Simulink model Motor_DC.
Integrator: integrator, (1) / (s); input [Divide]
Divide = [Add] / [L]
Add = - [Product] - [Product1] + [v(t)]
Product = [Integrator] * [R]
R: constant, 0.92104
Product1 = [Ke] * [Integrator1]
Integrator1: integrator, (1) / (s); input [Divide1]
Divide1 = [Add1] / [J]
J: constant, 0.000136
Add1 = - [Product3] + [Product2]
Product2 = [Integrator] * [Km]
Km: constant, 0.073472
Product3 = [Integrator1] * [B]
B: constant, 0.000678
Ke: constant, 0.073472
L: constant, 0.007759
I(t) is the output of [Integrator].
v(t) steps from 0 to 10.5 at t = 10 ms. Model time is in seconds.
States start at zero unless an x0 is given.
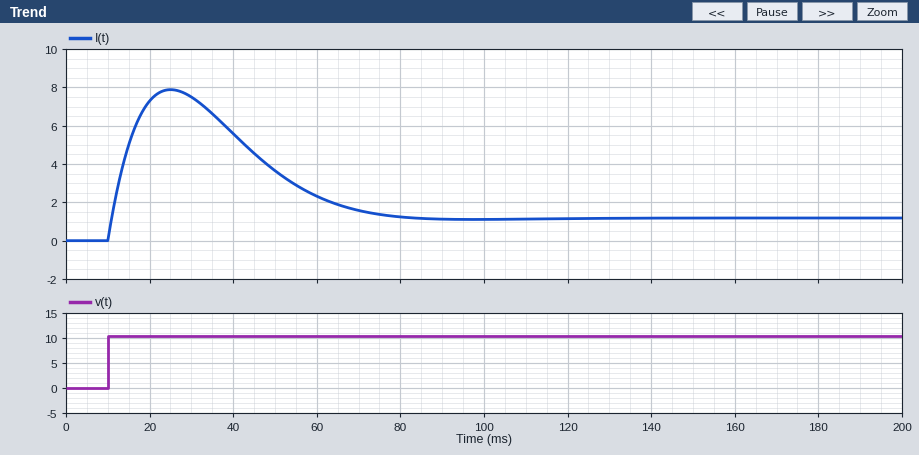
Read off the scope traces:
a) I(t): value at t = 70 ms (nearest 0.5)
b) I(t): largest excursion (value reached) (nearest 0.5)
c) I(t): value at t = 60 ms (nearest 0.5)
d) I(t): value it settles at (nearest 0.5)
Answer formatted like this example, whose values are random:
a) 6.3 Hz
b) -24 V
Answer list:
a) 1.5
b) 8.0
c) 2.5
d) 1.0
